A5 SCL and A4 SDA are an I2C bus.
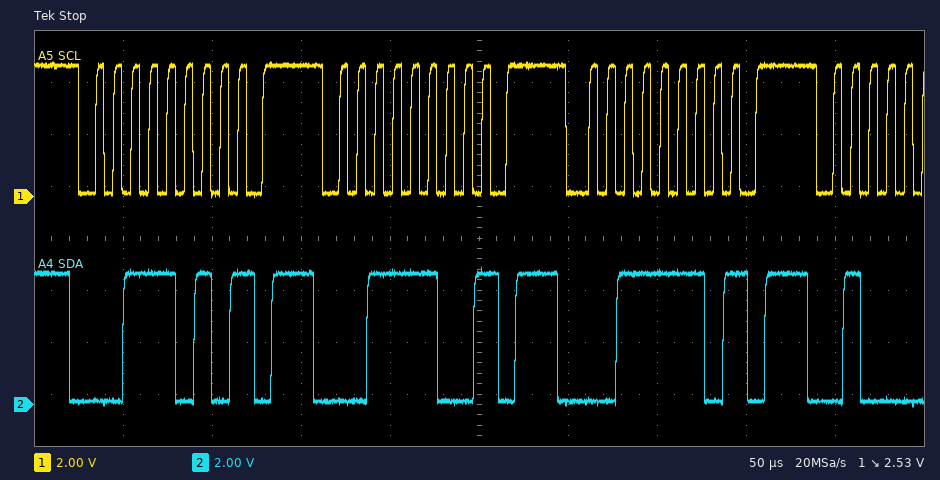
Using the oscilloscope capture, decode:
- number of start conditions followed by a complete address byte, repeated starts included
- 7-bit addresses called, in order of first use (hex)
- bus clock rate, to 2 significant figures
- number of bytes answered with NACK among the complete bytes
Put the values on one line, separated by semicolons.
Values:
3; 0x1D 0x1E 0x1F; 100 kHz; 3
